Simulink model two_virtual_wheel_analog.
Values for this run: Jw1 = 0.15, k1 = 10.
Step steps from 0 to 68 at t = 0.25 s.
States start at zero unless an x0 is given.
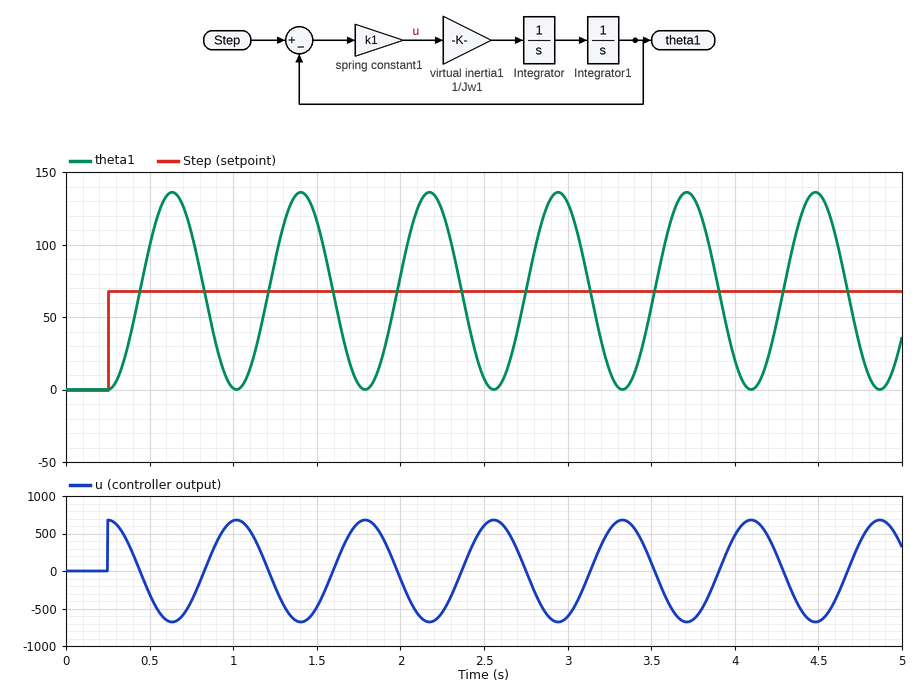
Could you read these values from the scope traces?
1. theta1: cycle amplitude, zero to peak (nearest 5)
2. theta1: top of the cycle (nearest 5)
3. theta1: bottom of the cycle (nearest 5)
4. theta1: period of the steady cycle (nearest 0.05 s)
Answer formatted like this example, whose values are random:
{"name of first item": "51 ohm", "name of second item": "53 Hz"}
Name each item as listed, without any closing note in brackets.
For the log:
{"theta1: cycle amplitude, zero to peak": "70", "theta1: top of the cycle": "135", "theta1: bottom of the cycle": "0", "theta1: period of the steady cycle": "0.75 s"}
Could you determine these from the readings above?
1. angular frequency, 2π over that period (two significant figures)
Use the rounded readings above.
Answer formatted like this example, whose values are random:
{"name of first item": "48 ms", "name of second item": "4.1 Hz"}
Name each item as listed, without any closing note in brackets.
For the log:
{"angular frequency, 2π over that period": "8.4 rad/s"}
